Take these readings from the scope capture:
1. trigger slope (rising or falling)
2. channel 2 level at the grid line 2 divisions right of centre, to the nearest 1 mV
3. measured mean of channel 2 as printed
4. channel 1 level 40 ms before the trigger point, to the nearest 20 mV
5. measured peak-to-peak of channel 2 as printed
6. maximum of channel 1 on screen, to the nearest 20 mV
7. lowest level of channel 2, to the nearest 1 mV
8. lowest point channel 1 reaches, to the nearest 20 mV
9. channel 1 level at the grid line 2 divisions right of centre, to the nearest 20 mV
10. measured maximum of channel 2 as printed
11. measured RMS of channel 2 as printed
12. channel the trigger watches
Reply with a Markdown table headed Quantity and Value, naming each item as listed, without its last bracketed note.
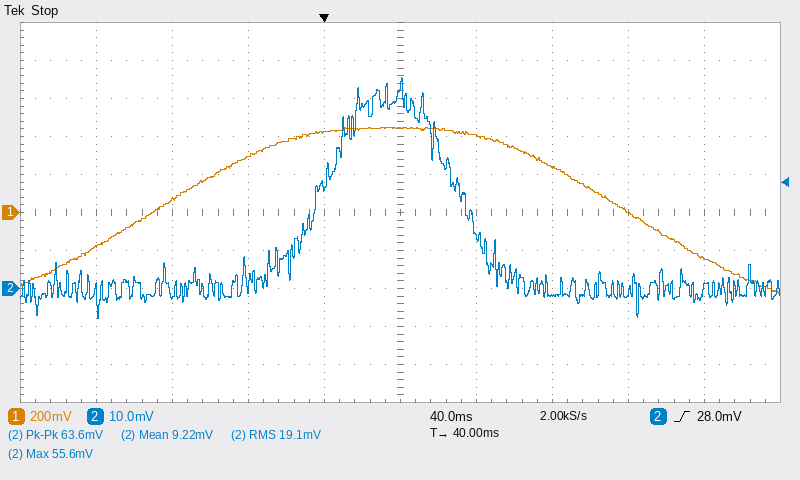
| Quantity | Value |
|---|---|
| trigger slope | rising |
| channel 2 level at the grid line 2 divisions right of centre, to the nearest 1 mV | -2 mV |
| measured mean of channel 2 as printed | 9.22 mV |
| channel 1 level 40 ms before the trigger point, to the nearest 20 mV | 300 mV |
| measured peak-to-peak of channel 2 as printed | 63.6 mV |
| maximum of channel 1 on screen, to the nearest 20 mV | 440 mV |
| lowest level of channel 2, to the nearest 1 mV | -8 mV |
| lowest point channel 1 reaches, to the nearest 20 mV | -420 mV |
| channel 1 level at the grid line 2 divisions right of centre, to the nearest 20 mV | 240 mV |
| measured maximum of channel 2 as printed | 55.6 mV |
| measured RMS of channel 2 as printed | 19.1 mV |
| channel the trigger watches | channel 2 |
